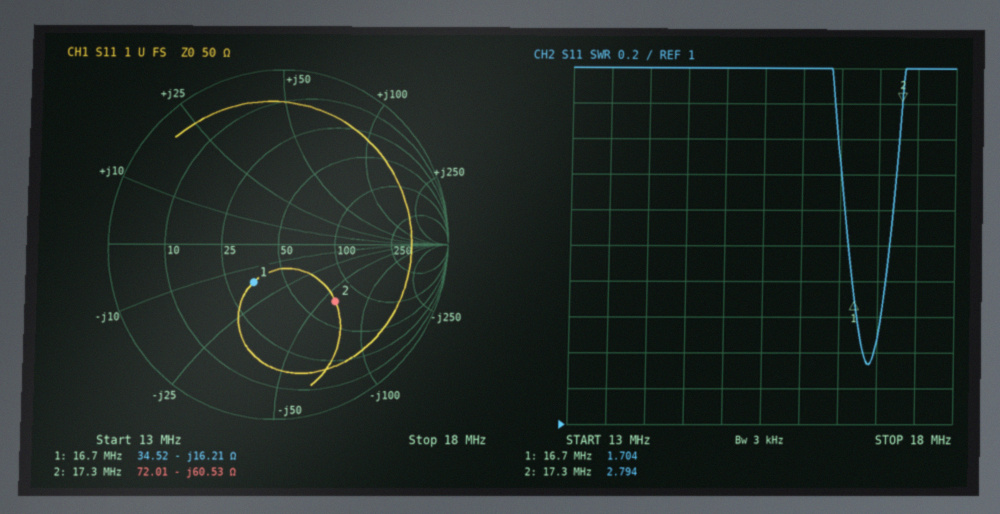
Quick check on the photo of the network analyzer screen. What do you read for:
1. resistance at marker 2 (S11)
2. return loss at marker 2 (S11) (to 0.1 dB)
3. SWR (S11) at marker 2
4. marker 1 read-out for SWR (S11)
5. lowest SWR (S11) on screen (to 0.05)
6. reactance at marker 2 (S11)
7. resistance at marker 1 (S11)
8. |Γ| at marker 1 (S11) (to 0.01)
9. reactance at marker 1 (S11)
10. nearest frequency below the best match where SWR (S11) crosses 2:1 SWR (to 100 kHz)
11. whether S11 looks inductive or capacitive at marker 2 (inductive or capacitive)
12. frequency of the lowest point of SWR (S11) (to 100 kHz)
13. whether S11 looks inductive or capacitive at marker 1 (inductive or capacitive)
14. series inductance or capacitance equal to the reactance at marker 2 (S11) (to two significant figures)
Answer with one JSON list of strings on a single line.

["72.01 Ω", "6.5 dB", "2.794", "1.704", "1.35", "-60.53 Ω", "34.52 Ω", "0.26", "-16.21 Ω", "16.6 MHz", "capacitive", "16.9 MHz", "capacitive", "150 pF"]
